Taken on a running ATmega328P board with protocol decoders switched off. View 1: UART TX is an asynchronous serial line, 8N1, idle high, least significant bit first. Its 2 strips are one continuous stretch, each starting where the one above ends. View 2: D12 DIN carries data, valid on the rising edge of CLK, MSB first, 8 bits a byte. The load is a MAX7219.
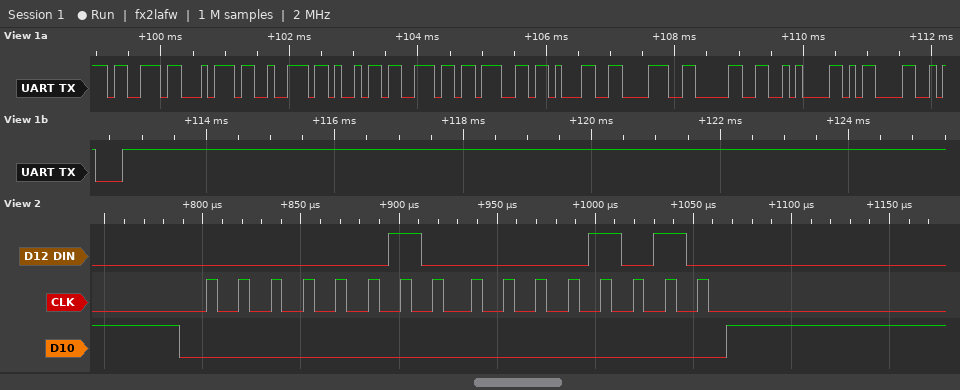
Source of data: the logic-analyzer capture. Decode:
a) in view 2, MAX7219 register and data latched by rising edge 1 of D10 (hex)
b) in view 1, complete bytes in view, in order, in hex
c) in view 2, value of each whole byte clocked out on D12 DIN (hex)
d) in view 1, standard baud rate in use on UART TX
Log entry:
register 0x2, data 0x0A
73 74 72 69 6E 67 31 38 30 0A 0D 0A
02 0A
9600 baud
